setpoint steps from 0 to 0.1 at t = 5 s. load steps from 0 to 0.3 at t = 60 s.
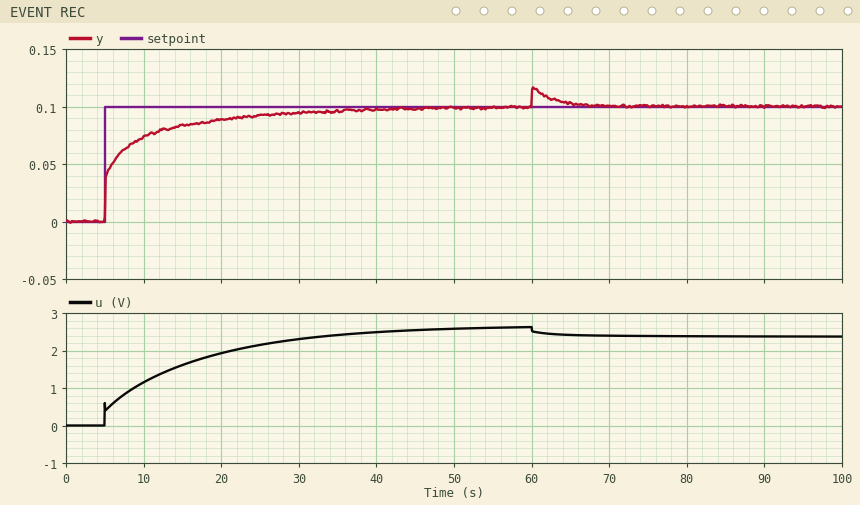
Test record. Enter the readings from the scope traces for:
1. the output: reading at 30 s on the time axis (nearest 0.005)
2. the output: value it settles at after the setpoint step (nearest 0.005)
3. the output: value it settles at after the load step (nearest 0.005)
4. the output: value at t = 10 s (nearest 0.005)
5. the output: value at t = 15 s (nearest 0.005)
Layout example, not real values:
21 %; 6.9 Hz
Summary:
0.095; 0.100; 0.100; 0.075; 0.085
